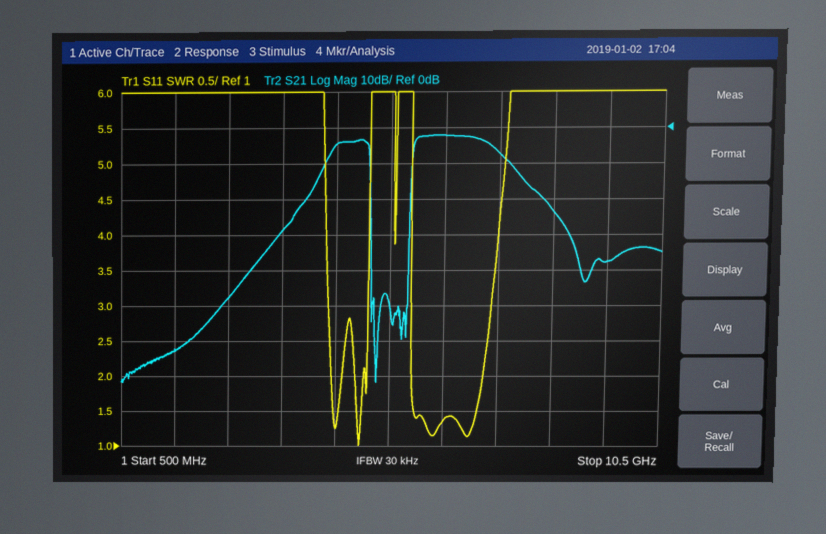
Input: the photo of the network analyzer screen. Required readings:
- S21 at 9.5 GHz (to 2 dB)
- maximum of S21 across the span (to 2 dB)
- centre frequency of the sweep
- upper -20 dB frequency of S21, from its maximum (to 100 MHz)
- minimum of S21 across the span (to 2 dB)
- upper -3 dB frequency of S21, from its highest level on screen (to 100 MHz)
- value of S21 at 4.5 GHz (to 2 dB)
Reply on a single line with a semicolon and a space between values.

-38 dB; -2 dB; 5.5 GHz; 8.4 GHz; -72 dB; 7.3 GHz; -4 dB
